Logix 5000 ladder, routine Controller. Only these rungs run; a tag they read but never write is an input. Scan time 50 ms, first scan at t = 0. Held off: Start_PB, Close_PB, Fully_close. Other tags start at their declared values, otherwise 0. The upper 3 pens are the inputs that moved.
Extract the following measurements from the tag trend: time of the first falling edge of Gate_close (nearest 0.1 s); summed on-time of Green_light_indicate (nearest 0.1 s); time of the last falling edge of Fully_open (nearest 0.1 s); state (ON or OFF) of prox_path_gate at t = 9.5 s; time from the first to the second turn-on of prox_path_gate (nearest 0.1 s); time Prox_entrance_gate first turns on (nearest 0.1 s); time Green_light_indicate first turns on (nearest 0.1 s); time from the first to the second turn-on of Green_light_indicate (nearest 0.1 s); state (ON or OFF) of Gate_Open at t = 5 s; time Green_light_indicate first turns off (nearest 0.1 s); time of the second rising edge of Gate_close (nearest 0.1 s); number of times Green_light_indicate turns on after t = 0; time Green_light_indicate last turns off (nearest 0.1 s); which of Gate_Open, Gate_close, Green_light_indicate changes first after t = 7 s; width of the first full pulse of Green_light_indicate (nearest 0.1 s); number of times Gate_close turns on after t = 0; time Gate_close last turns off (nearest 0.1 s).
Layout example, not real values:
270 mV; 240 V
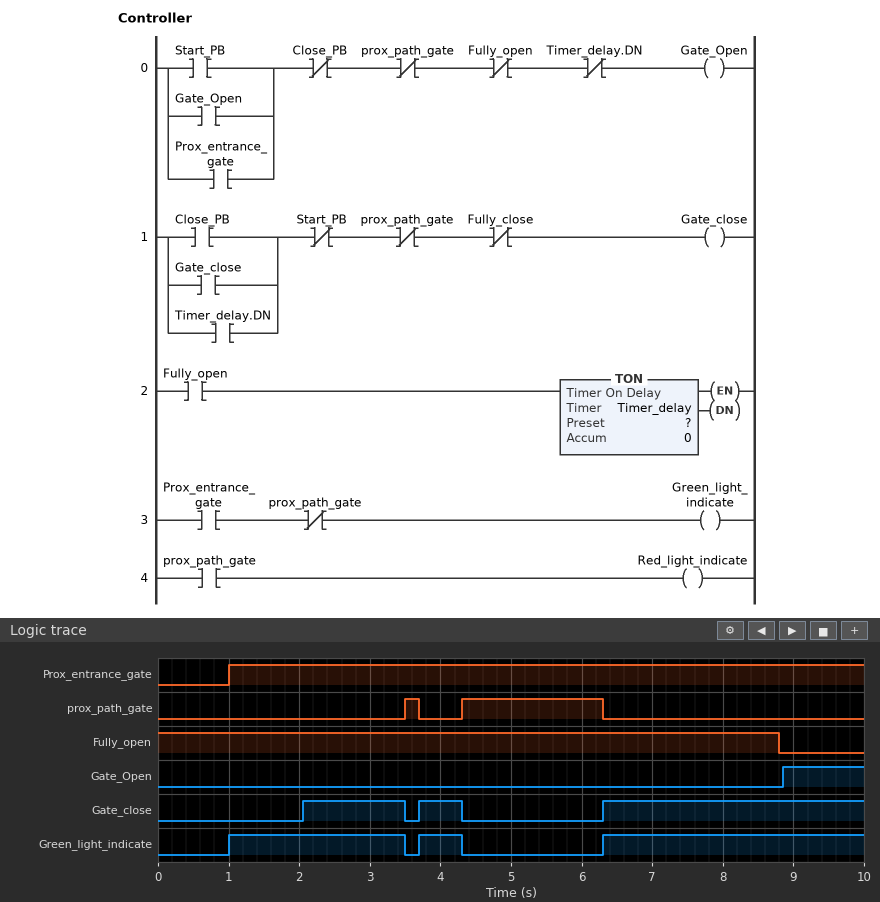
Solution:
3.5 s; 6.8 s; 8.8 s; OFF; 0.8 s; 1.0 s; 1.0 s; 2.7 s; OFF; 3.5 s; 3.7 s; 3; 4.3 s; Gate_Open; 2.5 s; 3; 4.3 s
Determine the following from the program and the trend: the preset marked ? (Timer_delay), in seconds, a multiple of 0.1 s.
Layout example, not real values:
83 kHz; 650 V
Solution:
2.0 s
